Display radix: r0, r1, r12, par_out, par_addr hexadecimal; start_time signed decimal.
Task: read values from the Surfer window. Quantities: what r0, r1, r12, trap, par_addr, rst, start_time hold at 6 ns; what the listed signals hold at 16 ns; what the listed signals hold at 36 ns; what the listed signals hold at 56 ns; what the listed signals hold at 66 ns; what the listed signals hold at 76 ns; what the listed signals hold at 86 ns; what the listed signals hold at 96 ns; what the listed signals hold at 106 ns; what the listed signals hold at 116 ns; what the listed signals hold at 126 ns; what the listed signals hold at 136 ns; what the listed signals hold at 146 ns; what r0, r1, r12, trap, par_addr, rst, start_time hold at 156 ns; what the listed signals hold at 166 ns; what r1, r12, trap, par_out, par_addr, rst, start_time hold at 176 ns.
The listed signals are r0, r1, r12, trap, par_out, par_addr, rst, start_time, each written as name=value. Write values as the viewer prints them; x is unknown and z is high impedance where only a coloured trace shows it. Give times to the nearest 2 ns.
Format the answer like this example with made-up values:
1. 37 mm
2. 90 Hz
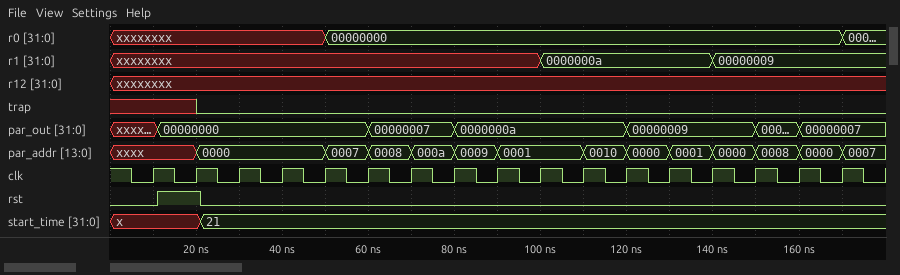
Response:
1. r0=xxxxxxxx, r1=xxxxxxxx, r12=xxxxxxxx, trap=x, par_addr=xxxx, rst=0, start_time=x
2. r0=xxxxxxxx, r1=xxxxxxxx, r12=xxxxxxxx, trap=x, par_out=00000000, par_addr=xxxx, rst=1, start_time=x
3. r0=xxxxxxxx, r1=xxxxxxxx, r12=xxxxxxxx, trap=0, par_out=00000000, par_addr=0000, rst=0, start_time=21
4. r0=00000000, r1=xxxxxxxx, r12=xxxxxxxx, trap=0, par_out=00000000, par_addr=0007, rst=0, start_time=21
5. r0=00000000, r1=xxxxxxxx, r12=xxxxxxxx, trap=0, par_out=00000007, par_addr=0008, rst=0, start_time=21
6. r0=00000000, r1=xxxxxxxx, r12=xxxxxxxx, trap=0, par_out=00000007, par_addr=000a, rst=0, start_time=21
7. r0=00000000, r1=xxxxxxxx, r12=xxxxxxxx, trap=0, par_out=0000000a, par_addr=0009, rst=0, start_time=21
8. r0=00000000, r1=xxxxxxxx, r12=xxxxxxxx, trap=0, par_out=0000000a, par_addr=0001, rst=0, start_time=21
9. r0=00000000, r1=0000000a, r12=xxxxxxxx, trap=0, par_out=0000000a, par_addr=0001, rst=0, start_time=21
10. r0=00000000, r1=0000000a, r12=xxxxxxxx, trap=0, par_out=0000000a, par_addr=0010, rst=0, start_time=21
11. r0=00000000, r1=0000000a, r12=xxxxxxxx, trap=0, par_out=00000009, par_addr=0000, rst=0, start_time=21
12. r0=00000000, r1=0000000a, r12=xxxxxxxx, trap=0, par_out=00000009, par_addr=0001, rst=0, start_time=21
13. r0=00000000, r1=00000009, r12=xxxxxxxx, trap=0, par_out=00000009, par_addr=0000, rst=0, start_time=21
14. r0=00000000, r1=00000009, r12=xxxxxxxx, trap=0, par_addr=0008, rst=0, start_time=21
15. r0=00000000, r1=00000009, r12=xxxxxxxx, trap=0, par_out=00000007, par_addr=0000, rst=0, start_time=21
16. r1=00000009, r12=xxxxxxxx, trap=0, par_out=00000007, par_addr=0007, rst=0, start_time=21
